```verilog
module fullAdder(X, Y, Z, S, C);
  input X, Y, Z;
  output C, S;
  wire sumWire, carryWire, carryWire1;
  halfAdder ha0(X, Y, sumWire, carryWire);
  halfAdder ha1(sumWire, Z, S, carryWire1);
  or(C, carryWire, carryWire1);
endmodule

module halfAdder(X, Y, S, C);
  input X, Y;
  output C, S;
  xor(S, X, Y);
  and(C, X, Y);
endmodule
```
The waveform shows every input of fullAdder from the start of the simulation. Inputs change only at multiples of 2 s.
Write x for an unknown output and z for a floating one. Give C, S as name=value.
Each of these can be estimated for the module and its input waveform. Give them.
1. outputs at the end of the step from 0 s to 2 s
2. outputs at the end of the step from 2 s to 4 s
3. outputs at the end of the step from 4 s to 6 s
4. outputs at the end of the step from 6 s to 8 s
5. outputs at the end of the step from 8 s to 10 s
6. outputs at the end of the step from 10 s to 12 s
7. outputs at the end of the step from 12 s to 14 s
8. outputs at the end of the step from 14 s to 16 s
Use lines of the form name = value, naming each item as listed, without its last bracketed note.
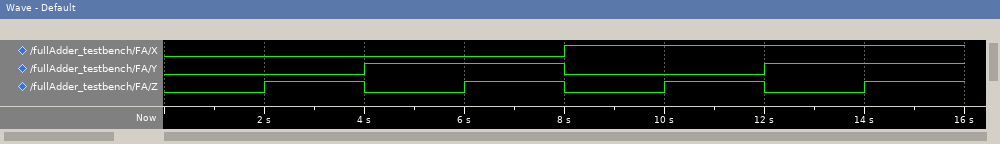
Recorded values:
outputs at the end of the step from 0 s to 2 s = C=0, S=0
outputs at the end of the step from 2 s to 4 s = C=0, S=1
outputs at the end of the step from 4 s to 6 s = C=0, S=1
outputs at the end of the step from 6 s to 8 s = C=1, S=0
outputs at the end of the step from 8 s to 10 s = C=0, S=1
outputs at the end of the step from 10 s to 12 s = C=1, S=0
outputs at the end of the step from 12 s to 14 s = C=1, S=0
outputs at the end of the step from 14 s to 16 s = C=1, S=1
